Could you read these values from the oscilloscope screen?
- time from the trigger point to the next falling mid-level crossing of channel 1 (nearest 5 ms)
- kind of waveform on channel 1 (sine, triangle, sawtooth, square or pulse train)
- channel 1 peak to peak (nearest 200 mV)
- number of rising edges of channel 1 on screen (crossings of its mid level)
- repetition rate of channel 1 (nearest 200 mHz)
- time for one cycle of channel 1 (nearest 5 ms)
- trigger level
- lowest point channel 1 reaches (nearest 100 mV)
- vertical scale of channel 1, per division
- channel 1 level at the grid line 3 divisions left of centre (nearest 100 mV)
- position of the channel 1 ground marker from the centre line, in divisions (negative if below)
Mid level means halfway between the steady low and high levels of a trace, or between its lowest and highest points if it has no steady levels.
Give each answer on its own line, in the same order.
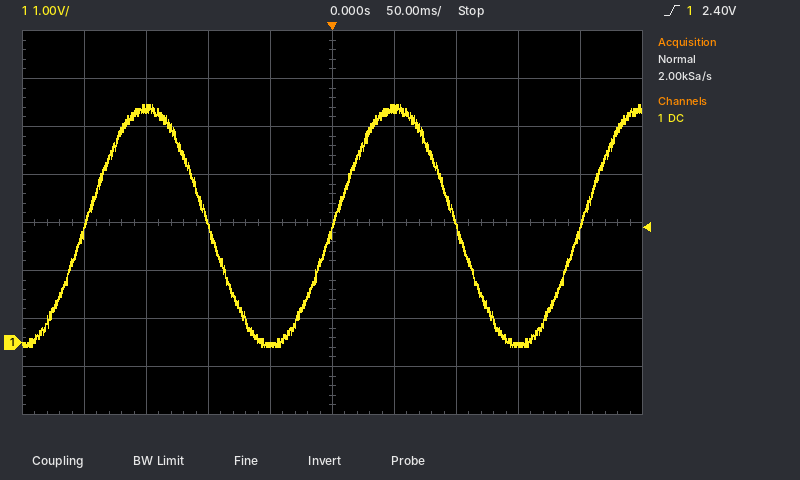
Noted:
100 ms
sine
5.0 V
3
5.0 Hz
200 ms
2.40 V
-100 mV
1 V
4.9 V
-2.5 div
